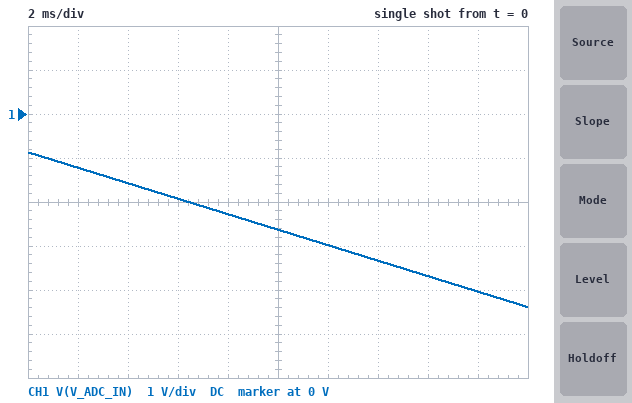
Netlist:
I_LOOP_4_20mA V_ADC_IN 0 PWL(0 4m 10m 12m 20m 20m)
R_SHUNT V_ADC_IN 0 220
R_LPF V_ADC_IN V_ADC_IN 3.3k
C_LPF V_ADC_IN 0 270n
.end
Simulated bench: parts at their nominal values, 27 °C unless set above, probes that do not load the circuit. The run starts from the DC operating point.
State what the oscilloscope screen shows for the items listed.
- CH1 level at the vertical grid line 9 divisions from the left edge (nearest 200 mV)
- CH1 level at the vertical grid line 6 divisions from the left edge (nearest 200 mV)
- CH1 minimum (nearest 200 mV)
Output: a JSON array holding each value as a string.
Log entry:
["-4.0 V", "-3.0 V", "-4.4 V"]
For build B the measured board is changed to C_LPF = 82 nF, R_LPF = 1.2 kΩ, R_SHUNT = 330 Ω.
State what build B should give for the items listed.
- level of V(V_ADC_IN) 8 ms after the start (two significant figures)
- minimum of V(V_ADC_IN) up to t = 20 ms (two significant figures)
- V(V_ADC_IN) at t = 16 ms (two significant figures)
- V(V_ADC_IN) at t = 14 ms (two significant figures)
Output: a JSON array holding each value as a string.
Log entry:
["-3.4 V", "-6.6 V", "-5.5 V", "-5.0 V"]
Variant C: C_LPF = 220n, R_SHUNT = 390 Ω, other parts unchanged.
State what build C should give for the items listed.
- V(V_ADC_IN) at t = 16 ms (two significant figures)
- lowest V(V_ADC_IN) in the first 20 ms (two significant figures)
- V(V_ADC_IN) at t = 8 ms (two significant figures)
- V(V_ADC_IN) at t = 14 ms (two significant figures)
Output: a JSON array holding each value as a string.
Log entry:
["-6.5 V", "-7.8 V", "-4.0 V", "-5.9 V"]
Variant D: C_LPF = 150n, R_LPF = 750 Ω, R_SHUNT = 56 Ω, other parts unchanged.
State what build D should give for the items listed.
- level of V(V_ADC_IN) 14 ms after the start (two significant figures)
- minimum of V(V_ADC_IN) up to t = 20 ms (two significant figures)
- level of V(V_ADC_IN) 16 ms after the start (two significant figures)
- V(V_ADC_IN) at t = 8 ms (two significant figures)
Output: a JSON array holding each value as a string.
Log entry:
["-850 mV", "-1.1 V", "-940 mV", "-580 mV"]
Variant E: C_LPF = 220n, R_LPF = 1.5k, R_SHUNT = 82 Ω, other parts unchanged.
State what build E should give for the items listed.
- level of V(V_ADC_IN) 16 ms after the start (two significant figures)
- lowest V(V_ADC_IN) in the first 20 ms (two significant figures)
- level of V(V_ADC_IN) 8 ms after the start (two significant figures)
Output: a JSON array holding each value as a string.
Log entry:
["-1.4 V", "-1.6 V", "-850 mV"]
